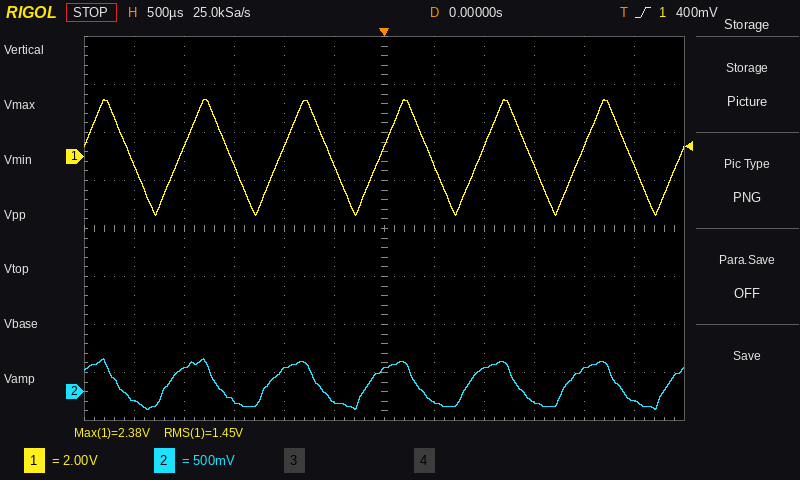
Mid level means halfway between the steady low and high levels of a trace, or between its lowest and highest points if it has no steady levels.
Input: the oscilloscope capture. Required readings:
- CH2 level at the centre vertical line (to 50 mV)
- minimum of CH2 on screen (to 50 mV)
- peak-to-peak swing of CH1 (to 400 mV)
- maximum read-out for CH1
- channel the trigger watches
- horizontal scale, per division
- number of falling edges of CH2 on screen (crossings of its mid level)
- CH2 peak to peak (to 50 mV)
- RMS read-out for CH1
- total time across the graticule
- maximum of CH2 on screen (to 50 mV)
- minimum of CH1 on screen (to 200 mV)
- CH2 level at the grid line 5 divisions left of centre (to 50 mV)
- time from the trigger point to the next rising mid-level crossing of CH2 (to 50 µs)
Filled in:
250 mV
-200 mV
4.8 V
2.38 V
CH1
500 µs
6
550 mV
1.45 V
6 ms
350 mV
-2.4 V
-100 mV
850 µs
